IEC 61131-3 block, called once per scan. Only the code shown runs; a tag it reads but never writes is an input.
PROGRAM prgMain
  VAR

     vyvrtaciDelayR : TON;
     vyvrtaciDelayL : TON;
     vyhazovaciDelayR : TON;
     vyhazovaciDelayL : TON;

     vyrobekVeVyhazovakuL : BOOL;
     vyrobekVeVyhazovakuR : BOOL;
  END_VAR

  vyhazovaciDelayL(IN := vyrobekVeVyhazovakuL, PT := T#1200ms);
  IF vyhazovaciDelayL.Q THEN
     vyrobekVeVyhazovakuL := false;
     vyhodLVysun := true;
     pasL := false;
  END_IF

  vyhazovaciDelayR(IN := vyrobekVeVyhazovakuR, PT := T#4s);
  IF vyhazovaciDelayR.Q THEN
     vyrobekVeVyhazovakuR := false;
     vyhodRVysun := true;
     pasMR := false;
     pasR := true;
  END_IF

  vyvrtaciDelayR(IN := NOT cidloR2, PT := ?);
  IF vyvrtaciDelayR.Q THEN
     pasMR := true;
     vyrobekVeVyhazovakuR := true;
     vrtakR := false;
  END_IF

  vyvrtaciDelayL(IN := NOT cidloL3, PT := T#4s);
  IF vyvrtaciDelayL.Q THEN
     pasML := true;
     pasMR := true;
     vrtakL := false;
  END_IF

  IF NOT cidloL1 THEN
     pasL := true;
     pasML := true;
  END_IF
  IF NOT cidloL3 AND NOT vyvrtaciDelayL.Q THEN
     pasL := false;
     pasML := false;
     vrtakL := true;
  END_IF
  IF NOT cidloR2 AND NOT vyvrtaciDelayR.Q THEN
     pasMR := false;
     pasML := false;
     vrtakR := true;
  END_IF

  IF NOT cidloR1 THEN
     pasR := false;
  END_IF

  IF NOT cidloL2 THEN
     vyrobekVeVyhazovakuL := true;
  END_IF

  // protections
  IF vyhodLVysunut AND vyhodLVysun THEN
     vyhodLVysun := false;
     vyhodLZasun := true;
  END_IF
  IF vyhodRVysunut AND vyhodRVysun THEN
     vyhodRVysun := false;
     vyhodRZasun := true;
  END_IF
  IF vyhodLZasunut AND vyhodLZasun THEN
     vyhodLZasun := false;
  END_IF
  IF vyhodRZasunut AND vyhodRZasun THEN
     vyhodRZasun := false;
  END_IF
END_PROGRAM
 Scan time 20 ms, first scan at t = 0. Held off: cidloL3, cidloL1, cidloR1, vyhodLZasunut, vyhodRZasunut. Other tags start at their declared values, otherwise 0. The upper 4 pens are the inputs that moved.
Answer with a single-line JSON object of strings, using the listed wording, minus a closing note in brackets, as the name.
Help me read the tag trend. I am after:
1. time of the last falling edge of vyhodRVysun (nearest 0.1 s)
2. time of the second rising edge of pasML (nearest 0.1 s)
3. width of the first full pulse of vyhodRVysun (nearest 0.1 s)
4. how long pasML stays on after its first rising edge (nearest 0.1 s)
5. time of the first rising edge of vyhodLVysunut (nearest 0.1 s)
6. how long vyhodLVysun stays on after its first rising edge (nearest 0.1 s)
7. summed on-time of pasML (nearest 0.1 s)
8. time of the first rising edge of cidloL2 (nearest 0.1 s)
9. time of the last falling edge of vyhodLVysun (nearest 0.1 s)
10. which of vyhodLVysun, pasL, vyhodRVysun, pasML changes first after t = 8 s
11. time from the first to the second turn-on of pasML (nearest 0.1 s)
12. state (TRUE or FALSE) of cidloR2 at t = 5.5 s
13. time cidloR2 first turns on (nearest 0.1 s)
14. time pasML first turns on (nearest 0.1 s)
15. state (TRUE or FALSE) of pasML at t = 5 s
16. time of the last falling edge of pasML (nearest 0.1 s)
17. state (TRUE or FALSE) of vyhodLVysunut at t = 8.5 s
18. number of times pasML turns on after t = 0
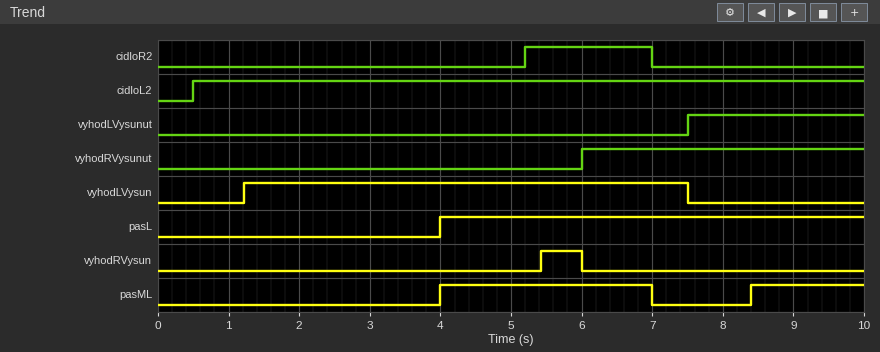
{"time of the last falling edge of vyhodRVysun": "6.0 s", "time of the second rising edge of pasML": "8.4 s", "width of the first full pulse of vyhodRVysun": "0.6 s", "how long pasML stays on after its first rising edge": "3.0 s", "time of the first rising edge of vyhodLVysunut": "7.5 s", "how long vyhodLVysun stays on after its first rising edge": "6.3 s", "summed on-time of pasML": "4.6 s", "time of the first rising edge of cidloL2": "0.5 s", "time of the last falling edge of vyhodLVysun": "7.5 s", "which of vyhodLVysun, pasL, vyhodRVysun, pasML changes first after t = 8 s": "pasML", "time from the first to the second turn-on of pasML": "4.4 s", "state (TRUE or FALSE) of cidloR2 at t = 5.5 s": "TRUE", "time cidloR2 first turns on": "5.2 s", "time pasML first turns on": "4.0 s", "state (TRUE or FALSE) of pasML at t = 5 s": "TRUE", "time of the last falling edge of pasML": "7.0 s", "state (TRUE or FALSE) of vyhodLVysunut at t = 8.5 s": "TRUE", "number of times pasML turns on after t = 0": "2"}
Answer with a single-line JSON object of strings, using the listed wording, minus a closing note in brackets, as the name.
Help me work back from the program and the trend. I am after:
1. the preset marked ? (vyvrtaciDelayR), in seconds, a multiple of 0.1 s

{"the preset marked ? (vyvrtaciDelayR), in seconds, a multiple of 0.1 s": "1.4 s"}
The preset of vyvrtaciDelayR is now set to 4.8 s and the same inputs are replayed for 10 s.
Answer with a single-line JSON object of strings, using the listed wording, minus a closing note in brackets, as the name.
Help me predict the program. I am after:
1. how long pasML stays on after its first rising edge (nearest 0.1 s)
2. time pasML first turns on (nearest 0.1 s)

{"how long pasML stays on after its first rising edge": "2.2 s", "time pasML first turns on": "4.8 s"}
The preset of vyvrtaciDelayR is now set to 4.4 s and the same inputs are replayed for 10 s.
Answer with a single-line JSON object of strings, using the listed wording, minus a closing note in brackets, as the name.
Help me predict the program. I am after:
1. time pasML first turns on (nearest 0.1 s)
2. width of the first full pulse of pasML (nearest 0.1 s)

{"time pasML first turns on": "4.4 s", "width of the first full pulse of pasML": "2.6 s"}
